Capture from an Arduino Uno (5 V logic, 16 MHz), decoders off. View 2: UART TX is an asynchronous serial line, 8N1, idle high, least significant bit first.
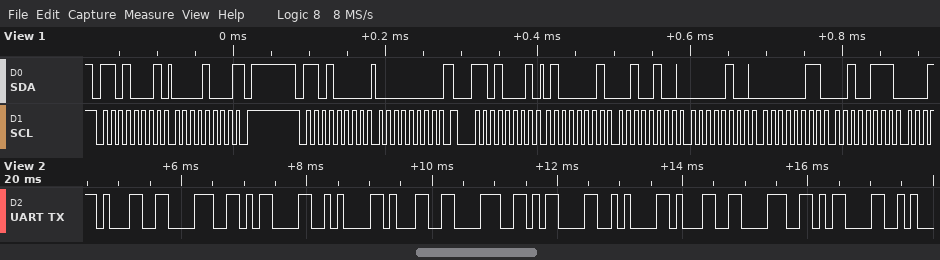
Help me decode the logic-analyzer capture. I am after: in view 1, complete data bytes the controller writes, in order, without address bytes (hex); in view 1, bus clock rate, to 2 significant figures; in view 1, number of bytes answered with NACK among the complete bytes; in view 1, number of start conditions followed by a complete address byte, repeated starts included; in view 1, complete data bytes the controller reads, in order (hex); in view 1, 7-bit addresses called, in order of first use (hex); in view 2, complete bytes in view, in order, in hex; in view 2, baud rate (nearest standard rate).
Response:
00
100 kHz
1
3
08 41 24 04 03 27
0x68
31 38 0D 0A 31 38 0D 0A 31 38 0D
9600 baud
